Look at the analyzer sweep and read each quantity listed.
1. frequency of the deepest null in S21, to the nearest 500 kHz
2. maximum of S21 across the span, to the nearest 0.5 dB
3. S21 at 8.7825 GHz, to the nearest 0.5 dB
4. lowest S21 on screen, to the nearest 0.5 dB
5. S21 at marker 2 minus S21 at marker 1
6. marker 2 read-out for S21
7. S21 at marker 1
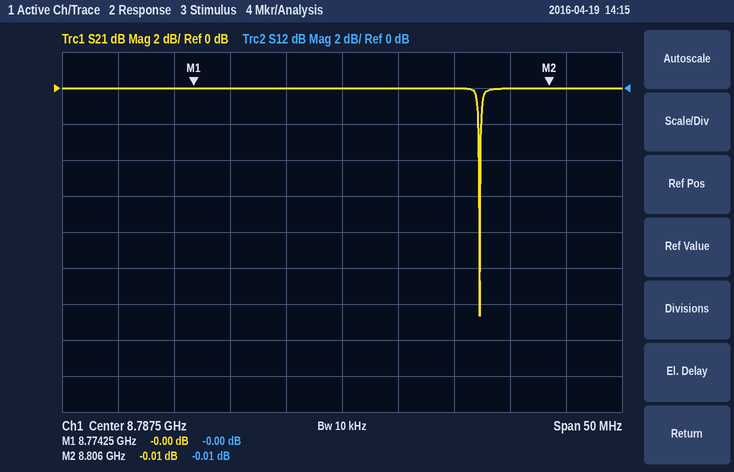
8.8000 GHz
0.0 dB
0.0 dB
-12.5 dB
-0.01 dB
-0.01 dB
-0.00 dB
